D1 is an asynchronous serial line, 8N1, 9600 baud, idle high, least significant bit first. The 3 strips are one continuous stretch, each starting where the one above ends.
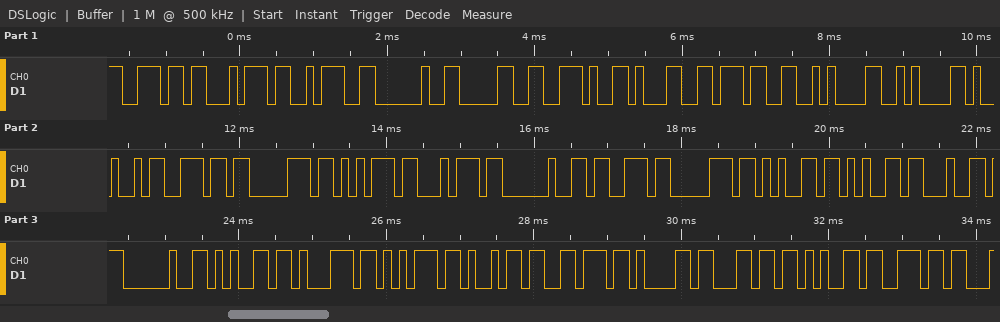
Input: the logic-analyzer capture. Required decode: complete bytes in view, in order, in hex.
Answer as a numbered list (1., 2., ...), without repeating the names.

1. 6E 74 3A 20 30 2E 31 37 0A 0A 49 6E 70 75 74 20 73 70 65 65 64 20 65 71 75 69 76 61 6C 65 6E
